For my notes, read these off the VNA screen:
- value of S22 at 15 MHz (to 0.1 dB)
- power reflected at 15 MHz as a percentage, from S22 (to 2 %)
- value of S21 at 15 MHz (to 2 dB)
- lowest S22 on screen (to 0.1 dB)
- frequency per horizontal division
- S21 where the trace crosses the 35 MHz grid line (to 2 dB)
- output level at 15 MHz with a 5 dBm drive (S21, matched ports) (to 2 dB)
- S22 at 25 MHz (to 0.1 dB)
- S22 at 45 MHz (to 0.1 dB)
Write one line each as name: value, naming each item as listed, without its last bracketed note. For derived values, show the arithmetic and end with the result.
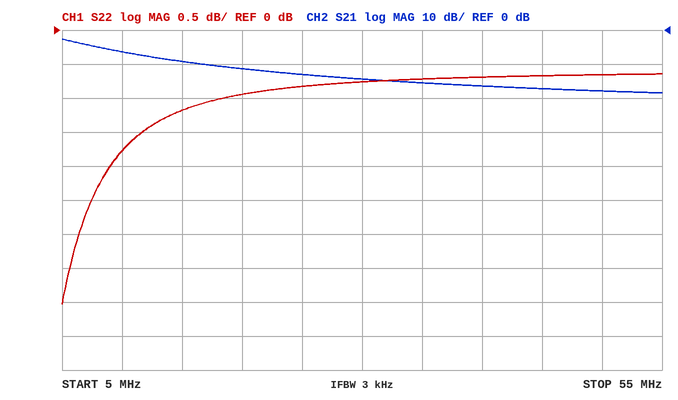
value of S22 at 15 MHz: -1.2 dB
power reflected at 15 MHz as a percentage, from S22: 10^(-1.2/10) ≈ 76 %
value of S21 at 15 MHz: -10 dB
lowest S22 on screen: -4.0 dB
frequency per horizontal division: 5 MHz
S21 where the trace crosses the 35 MHz grid line: -16 dB
output level at 15 MHz with a 5 dBm drive (S21, matched ports): 5 dBm + (-10 dB) = -4 dBm
S22 at 25 MHz: -0.8 dB
S22 at 45 MHz: -0.7 dB
